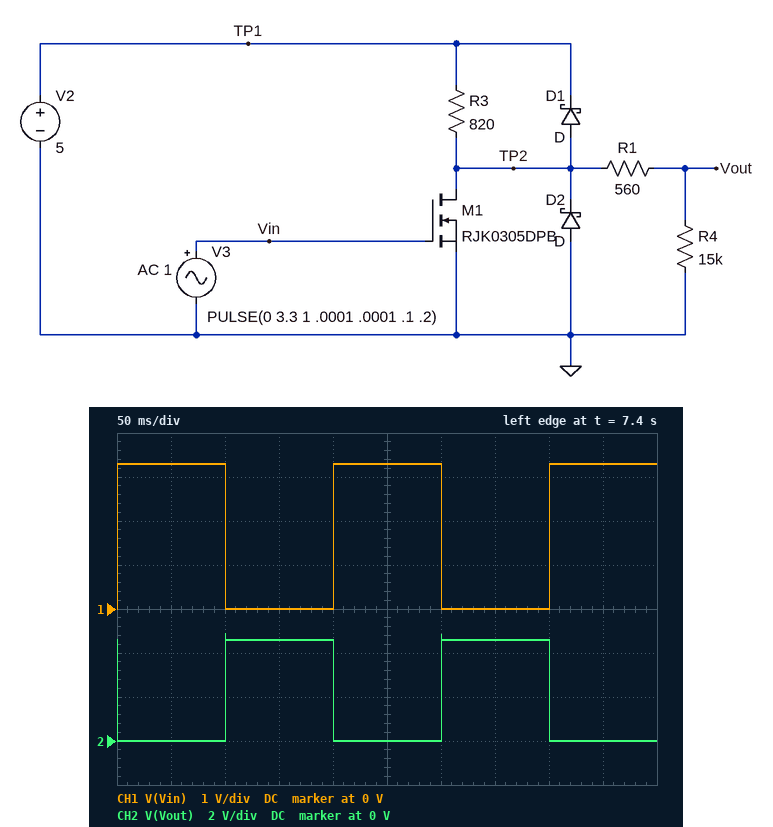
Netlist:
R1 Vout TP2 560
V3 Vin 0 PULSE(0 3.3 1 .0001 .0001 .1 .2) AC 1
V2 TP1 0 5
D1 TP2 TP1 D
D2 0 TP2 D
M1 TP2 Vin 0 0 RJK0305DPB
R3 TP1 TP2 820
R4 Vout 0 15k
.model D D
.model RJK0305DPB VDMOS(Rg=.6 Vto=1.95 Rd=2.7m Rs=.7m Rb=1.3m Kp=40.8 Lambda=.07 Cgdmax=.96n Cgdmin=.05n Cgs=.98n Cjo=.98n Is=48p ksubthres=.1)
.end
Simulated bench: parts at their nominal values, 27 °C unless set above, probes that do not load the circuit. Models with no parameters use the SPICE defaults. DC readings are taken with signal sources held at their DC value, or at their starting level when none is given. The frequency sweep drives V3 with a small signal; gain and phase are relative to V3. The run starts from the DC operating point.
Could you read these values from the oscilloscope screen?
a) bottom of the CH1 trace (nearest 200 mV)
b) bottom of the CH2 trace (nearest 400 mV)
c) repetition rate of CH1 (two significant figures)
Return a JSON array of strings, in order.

["0 V", "0 V", "5.0 Hz"]
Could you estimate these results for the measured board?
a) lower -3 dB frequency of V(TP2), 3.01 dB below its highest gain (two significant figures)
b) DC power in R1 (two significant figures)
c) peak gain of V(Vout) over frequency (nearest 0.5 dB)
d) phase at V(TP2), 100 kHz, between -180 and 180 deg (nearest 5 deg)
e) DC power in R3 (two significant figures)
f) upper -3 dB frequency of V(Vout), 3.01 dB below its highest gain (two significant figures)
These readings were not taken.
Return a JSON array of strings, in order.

["410 kHz", "52 µW", "-12.5 dB", "75 deg", "76 µW", "250 MHz"]
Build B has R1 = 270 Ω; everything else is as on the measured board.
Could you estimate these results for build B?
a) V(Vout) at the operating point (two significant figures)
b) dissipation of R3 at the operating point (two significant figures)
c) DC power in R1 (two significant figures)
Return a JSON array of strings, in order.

["4.7 V", "79 µW", "26 µW"]
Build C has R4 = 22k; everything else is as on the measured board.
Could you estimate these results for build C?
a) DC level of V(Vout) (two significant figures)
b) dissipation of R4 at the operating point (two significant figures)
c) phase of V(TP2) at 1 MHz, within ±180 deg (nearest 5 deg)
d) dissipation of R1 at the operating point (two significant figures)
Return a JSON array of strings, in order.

["4.7 V", "1.0 mW", "20 deg", "26 µW"]
